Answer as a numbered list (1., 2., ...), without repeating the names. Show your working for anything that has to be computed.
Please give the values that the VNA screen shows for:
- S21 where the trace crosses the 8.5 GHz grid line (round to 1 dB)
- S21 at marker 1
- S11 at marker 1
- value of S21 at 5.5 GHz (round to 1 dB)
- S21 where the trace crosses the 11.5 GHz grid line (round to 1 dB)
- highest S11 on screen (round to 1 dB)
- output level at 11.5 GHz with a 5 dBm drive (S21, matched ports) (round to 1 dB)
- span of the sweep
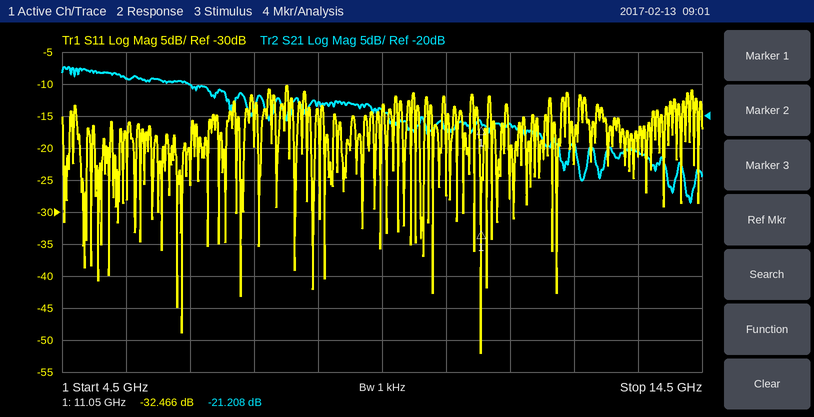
1. -18 dB
2. -21.208 dB
3. -32.466 dB
4. -14 dB
5. -21 dB
6. -10 dB
7. 5 dBm + (-21 dB) = -16 dBm
8. 10 GHz
